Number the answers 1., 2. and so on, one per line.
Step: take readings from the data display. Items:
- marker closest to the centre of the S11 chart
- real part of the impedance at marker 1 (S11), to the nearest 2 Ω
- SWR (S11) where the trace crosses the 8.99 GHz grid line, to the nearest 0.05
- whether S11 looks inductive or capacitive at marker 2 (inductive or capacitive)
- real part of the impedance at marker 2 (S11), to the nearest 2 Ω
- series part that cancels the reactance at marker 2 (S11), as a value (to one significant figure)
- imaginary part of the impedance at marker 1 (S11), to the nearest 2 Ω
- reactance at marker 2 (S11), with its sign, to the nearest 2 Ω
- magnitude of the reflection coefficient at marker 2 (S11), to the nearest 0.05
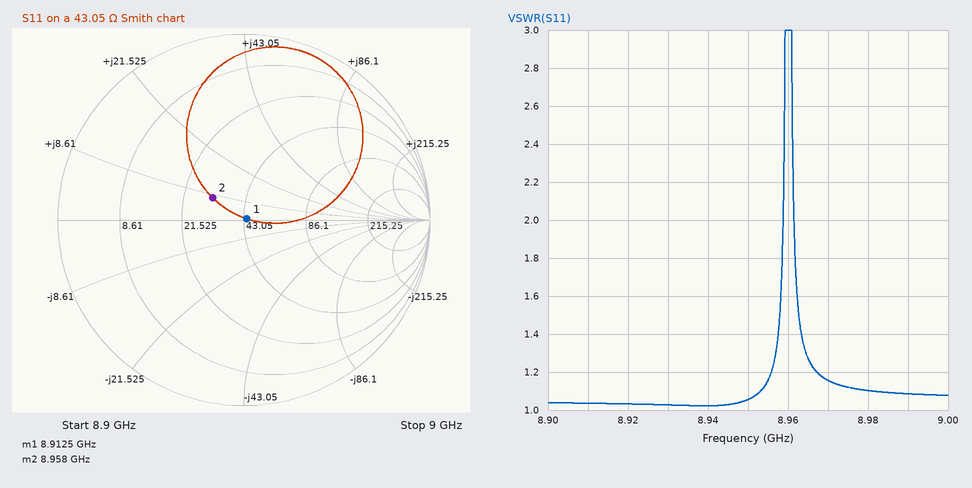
1. marker 1
2. 44 Ω
3. 1.10
4. inductive
5. 30 Ω
6. 2 pF
7. 0 Ω
8. +8 Ω
9. 0.20
